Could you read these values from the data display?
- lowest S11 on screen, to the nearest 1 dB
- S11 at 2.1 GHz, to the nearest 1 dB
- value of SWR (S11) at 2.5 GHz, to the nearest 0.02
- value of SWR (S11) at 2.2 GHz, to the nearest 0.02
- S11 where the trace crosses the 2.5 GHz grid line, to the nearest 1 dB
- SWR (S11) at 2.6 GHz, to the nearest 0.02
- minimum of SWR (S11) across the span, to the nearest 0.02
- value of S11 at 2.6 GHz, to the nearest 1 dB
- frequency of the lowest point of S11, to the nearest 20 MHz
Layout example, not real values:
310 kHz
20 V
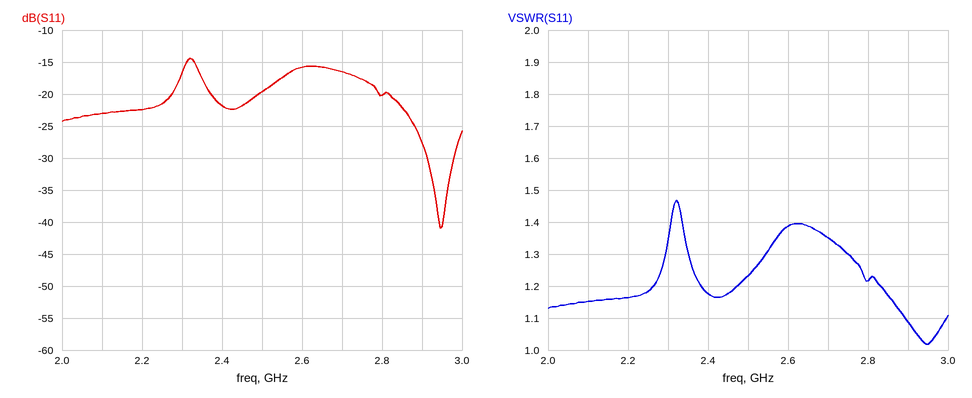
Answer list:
-41 dB
-23 dB
1.24
1.16
-20 dB
1.38
1.02
-16 dB
2.94 GHz
